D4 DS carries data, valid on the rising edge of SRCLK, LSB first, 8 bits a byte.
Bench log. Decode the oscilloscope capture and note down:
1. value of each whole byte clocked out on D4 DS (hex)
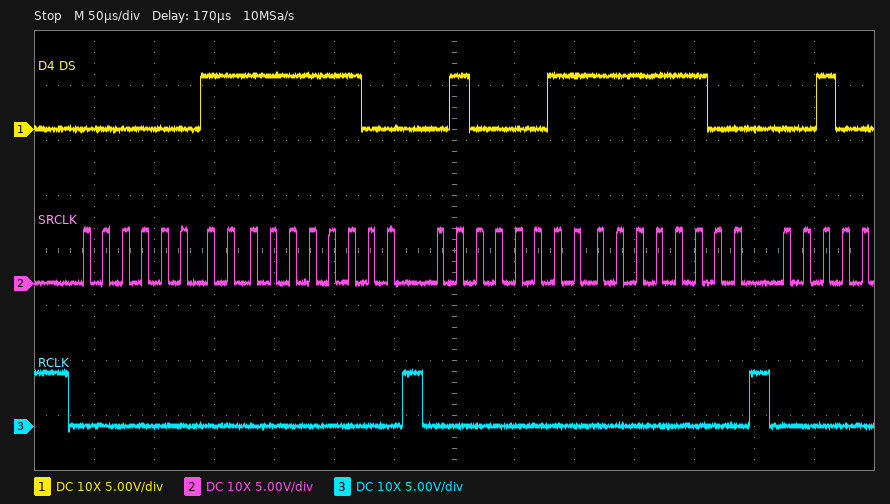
C0 3F C2 3F
